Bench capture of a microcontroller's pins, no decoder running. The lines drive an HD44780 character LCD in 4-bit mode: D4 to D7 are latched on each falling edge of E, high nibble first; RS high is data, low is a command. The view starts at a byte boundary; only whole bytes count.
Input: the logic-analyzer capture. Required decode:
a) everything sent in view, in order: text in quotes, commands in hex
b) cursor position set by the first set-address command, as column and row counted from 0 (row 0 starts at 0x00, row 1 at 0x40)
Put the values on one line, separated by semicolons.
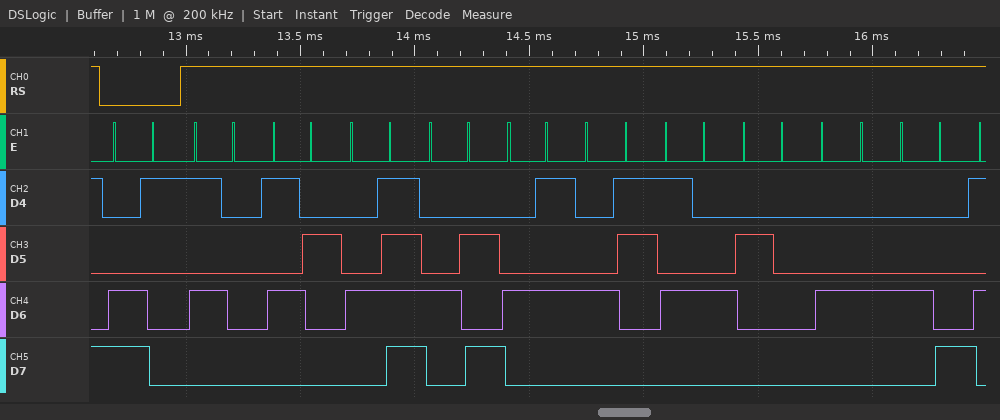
0xC1 "PROJECT DH"; column 1, row 1
